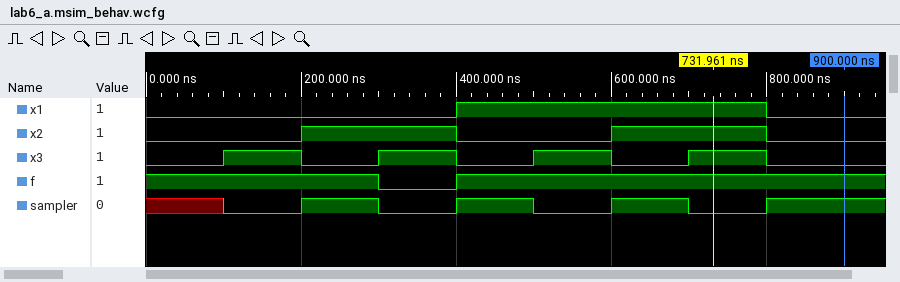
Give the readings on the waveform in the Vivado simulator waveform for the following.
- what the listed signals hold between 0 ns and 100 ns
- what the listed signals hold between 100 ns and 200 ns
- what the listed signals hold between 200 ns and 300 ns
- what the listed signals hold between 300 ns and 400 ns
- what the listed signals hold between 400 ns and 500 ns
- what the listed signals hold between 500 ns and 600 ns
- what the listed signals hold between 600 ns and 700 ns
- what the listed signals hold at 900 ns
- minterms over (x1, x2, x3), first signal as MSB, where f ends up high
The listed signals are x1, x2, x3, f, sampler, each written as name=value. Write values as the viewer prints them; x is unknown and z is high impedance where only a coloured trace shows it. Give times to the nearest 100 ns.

x1=0, x2=0, x3=0, f=1, sampler=x
x1=0, x2=0, x3=1, f=1, sampler=0
x1=0, x2=1, x3=0, f=1, sampler=1
x1=0, x2=1, x3=1, f=0, sampler=0
x1=1, x2=0, x3=0, f=1, sampler=1
x1=1, x2=0, x3=1, f=1, sampler=0
x1=1, x2=1, x3=0, f=1, sampler=1
x1=0, x2=0, x3=0, f=1, sampler=1
0, 1, 2, 4, 5, 6, 7
